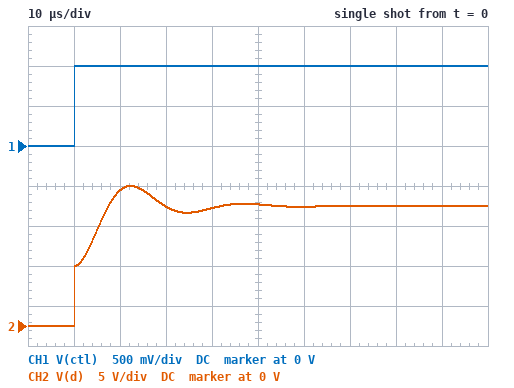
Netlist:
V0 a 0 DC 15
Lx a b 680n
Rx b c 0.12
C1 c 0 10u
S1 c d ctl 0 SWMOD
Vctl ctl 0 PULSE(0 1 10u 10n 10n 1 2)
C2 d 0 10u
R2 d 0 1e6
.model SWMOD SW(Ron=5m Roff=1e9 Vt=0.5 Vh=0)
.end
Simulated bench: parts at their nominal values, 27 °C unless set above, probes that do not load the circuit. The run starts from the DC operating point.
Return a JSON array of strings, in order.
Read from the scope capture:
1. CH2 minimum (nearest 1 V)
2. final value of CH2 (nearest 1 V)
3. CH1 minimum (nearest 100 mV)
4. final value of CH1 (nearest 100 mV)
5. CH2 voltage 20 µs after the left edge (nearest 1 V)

["0 V", "15 V", "0 V", "1.0 V", "17 V"]
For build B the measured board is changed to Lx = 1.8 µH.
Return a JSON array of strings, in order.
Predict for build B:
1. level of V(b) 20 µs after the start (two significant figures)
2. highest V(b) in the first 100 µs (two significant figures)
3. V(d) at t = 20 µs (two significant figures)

["16 V", "19 V", "14 V"]
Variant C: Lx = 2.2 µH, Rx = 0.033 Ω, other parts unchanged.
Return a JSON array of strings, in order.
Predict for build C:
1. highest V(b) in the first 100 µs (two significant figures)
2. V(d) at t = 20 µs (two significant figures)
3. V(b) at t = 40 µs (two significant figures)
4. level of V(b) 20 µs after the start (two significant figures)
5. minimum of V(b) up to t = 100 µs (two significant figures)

["21 V", "14 V", "16 V", "15 V", "7.5 V"]
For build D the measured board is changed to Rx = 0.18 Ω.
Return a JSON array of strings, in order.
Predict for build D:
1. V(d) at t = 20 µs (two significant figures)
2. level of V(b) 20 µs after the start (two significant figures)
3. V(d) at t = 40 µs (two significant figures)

["16 V", "17 V", "15 V"]
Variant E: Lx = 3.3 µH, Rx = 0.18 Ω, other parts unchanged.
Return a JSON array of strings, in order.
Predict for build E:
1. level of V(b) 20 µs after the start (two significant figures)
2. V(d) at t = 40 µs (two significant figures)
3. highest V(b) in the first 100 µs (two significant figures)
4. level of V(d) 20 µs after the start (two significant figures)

["14 V", "18 V", "19 V", "12 V"]
